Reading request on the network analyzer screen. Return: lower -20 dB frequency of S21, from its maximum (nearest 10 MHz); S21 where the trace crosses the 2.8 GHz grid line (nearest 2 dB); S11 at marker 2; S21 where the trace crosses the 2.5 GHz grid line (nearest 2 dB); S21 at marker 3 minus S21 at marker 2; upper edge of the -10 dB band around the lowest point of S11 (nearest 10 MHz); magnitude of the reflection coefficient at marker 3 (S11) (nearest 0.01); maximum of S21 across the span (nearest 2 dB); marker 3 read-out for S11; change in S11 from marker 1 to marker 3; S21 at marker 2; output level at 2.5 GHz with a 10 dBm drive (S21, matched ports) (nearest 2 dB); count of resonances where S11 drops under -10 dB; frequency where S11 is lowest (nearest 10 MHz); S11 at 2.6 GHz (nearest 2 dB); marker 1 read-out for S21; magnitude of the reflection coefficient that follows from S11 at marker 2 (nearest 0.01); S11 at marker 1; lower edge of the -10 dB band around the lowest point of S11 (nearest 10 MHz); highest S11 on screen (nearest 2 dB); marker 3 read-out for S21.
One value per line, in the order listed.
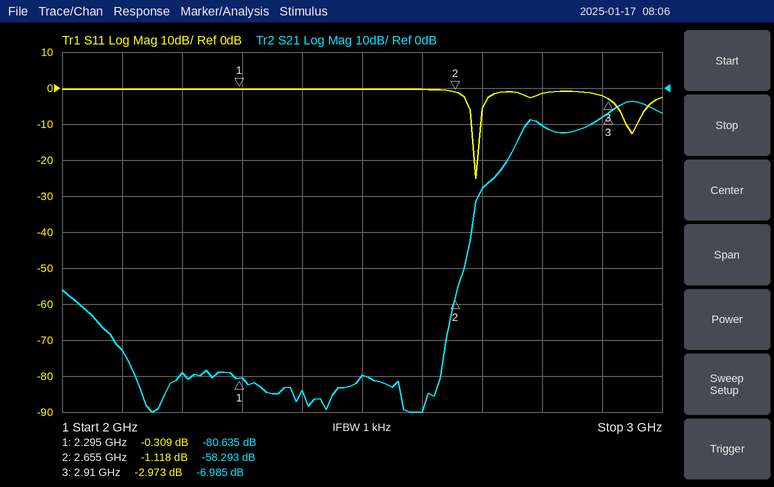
2.73 GHz
-10 dB
-1.118 dB
-80 dB
51.308 dB
2.70 GHz
0.71
-4 dB
-2.973 dB
-2.664 dB
-58.293 dB
-70 dBm
2
2.69 GHz
0 dB
-80.635 dB
0.88
-0.309 dB
2.68 GHz
0 dB
-6.985 dB
